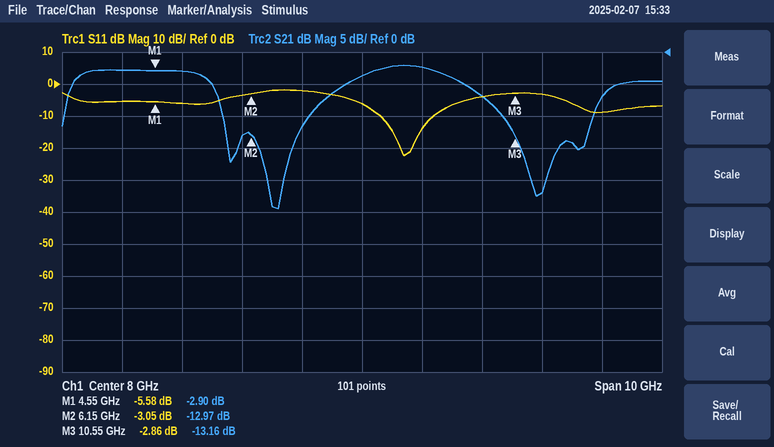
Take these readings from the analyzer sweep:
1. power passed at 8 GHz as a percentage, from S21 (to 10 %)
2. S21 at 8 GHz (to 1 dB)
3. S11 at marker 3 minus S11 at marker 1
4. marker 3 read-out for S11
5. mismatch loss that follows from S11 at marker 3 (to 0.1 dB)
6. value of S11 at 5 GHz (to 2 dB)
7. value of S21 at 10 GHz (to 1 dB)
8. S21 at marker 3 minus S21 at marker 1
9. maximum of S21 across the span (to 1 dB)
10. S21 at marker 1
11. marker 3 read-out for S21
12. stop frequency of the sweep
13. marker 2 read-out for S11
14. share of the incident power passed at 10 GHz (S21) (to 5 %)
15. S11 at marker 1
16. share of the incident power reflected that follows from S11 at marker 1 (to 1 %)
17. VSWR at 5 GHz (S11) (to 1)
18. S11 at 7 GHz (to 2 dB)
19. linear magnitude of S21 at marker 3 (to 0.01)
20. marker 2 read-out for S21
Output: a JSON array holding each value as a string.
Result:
["40 %", "-4 dB", "2.72 dB", "-2.86 dB", "3.2 dB", "-6 dB", "-7 dB", "-10.26 dB", "-2 dB", "-2.90 dB", "-13.16 dB", "13 GHz", "-3.05 dB", "20 %", "-5.58 dB", "28 %", "3", "-2 dB", "0.22", "-12.97 dB"]
